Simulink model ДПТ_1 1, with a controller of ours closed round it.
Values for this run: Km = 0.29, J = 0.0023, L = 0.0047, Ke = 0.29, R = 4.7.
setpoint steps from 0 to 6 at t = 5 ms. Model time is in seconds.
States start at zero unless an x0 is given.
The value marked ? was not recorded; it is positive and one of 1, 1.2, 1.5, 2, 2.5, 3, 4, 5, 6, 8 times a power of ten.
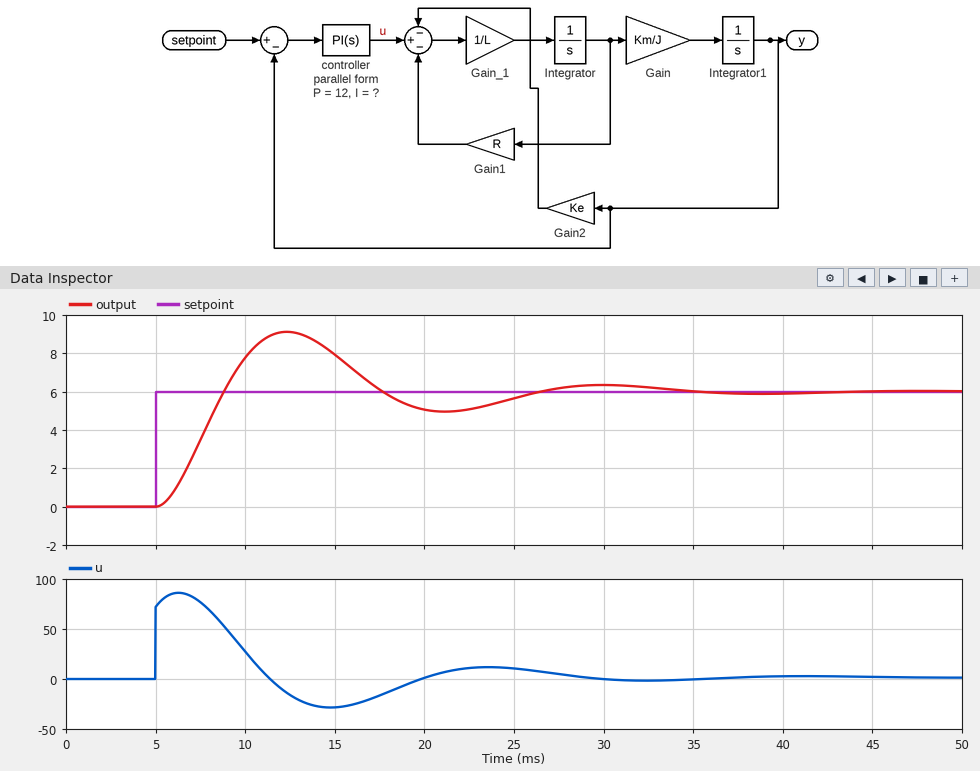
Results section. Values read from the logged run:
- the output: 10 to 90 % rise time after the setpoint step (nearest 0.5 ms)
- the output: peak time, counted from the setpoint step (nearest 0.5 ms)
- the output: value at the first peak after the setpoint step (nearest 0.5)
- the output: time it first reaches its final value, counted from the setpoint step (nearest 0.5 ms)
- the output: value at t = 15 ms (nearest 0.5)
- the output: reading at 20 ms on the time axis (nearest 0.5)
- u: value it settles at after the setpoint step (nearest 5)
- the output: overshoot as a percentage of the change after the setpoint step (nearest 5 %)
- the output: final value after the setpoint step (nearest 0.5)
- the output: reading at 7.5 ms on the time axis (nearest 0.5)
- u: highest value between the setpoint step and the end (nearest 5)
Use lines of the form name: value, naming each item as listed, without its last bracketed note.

the output: 10 to 90 % rise time after the setpoint step: 2.5 ms
the output: peak time, counted from the setpoint step: 7.5 ms
the output: value at the first peak after the setpoint step: 9.0
the output: time it first reaches its final value, counted from the setpoint step: 4.0 ms
the output: value at t = 15 ms: 8.0
the output: reading at 20 ms on the time axis: 5.0
u: value it settles at after the setpoint step: 0
the output: overshoot as a percentage of the change after the setpoint step: 50 %
the output: final value after the setpoint step: 6.0
the output: reading at 7.5 ms on the time axis: 3.5
u: highest value between the setpoint step and the end: 85
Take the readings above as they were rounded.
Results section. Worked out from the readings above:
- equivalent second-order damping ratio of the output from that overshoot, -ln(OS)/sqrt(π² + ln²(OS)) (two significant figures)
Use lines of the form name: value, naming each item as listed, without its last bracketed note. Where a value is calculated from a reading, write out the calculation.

equivalent second-order damping ratio of the output from that overshoot, -ln(OS)/sqrt(π² + ln²(OS)): ln(0.5) = -0.693; 0.693 / sqrt(9.870 + 0.480) = 0.22
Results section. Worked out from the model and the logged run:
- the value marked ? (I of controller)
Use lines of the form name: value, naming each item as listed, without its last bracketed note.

the value marked ?: 4000
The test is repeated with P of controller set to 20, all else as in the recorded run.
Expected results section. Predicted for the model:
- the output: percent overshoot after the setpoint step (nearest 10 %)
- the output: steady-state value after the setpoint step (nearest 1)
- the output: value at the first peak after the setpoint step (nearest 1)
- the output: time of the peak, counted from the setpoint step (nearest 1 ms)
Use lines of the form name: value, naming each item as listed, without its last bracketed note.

the output: percent overshoot after the setpoint step: 40 %
the output: steady-state value after the setpoint step: 6
the output: value at the first peak after the setpoint step: 8
the output: time of the peak, counted from the setpoint step: 6 ms
